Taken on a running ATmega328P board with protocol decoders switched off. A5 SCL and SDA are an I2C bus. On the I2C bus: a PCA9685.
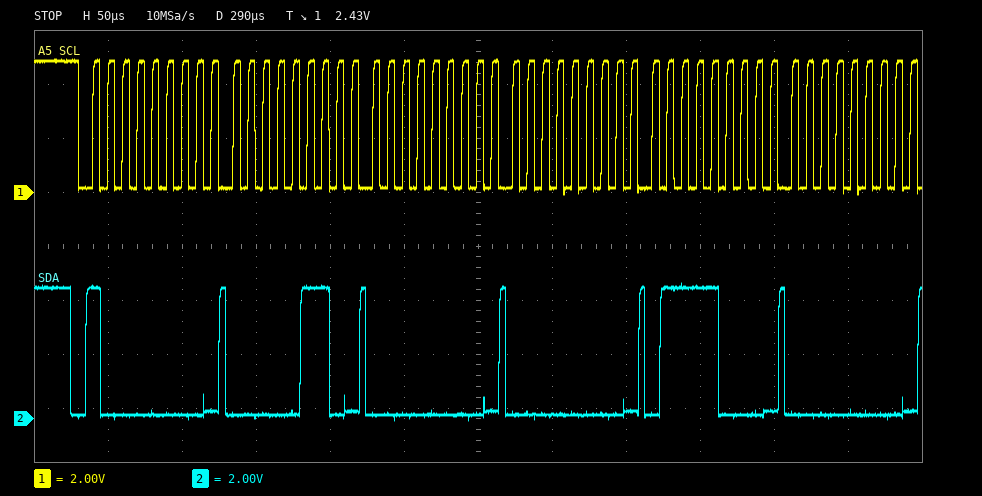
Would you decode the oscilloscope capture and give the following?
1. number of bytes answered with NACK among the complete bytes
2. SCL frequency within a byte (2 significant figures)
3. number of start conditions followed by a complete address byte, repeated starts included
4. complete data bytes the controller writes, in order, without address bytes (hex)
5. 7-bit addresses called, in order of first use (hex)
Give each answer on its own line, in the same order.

0
100 kHz
1
06 00 00 78 00
0x40
